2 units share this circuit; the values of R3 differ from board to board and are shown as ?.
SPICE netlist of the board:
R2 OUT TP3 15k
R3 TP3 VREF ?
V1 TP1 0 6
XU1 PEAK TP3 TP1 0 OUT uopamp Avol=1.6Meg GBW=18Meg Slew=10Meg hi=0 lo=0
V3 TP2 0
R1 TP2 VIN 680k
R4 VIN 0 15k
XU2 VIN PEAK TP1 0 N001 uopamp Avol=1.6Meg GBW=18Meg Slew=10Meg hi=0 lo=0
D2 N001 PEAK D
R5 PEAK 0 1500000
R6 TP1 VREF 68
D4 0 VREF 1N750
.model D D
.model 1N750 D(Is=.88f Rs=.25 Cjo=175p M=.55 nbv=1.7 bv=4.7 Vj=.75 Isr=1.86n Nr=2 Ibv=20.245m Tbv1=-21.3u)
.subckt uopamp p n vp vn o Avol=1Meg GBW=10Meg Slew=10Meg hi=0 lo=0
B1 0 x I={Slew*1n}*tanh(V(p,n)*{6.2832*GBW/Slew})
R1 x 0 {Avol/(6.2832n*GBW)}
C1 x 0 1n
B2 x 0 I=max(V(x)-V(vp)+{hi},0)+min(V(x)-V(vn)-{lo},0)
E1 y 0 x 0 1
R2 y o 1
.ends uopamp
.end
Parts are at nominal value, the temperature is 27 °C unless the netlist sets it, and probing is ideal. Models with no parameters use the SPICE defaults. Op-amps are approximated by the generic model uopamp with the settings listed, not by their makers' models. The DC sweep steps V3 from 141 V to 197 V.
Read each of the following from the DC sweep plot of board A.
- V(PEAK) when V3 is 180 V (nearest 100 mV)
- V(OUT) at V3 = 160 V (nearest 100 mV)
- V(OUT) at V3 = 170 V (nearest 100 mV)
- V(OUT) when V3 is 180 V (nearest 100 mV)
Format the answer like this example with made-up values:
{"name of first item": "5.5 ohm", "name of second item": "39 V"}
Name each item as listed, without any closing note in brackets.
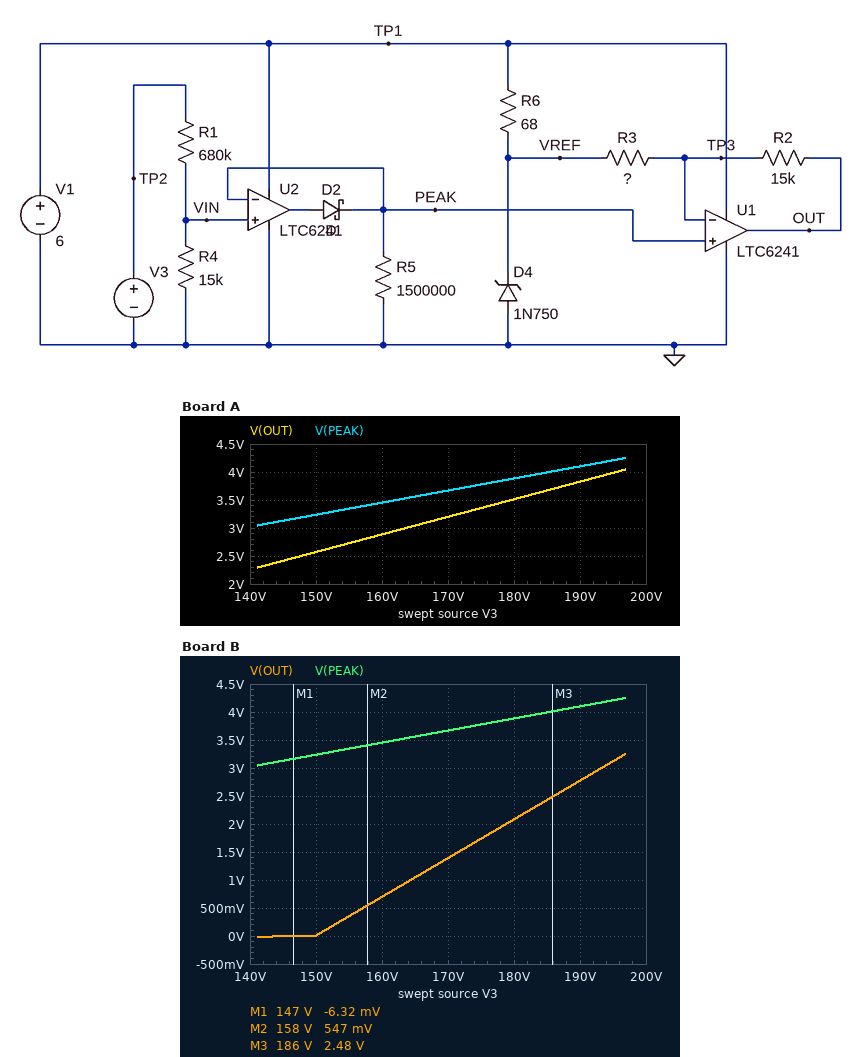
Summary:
{"V(PEAK) when V3 is 180 V": "3.9 V", "V(OUT) at V3 = 160 V": "2.9 V", "V(OUT) at V3 = 170 V": "3.2 V", "V(OUT) when V3 is 180 V": "3.5 V"}
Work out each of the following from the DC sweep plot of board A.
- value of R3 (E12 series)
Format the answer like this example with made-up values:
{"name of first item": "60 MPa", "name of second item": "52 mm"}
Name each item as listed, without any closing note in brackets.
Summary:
{"value of R3": "33 kΩ"}
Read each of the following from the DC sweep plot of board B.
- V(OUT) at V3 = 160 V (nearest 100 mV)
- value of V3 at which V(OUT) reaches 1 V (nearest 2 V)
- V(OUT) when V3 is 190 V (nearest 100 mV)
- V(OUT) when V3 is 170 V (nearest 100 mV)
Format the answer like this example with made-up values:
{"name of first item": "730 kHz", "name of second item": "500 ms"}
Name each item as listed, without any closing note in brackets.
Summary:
{"V(OUT) at V3 = 160 V": "700 mV", "value of V3 at which V(OUT) reaches 1 V": "164 V", "V(OUT) when V3 is 190 V": "2.8 V", "V(OUT) when V3 is 170 V": "1.4 V"}
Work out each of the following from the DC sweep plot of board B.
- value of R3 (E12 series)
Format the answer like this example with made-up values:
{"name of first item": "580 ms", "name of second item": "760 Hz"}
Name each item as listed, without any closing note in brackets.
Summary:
{"value of R3": "6.8 kΩ"}
